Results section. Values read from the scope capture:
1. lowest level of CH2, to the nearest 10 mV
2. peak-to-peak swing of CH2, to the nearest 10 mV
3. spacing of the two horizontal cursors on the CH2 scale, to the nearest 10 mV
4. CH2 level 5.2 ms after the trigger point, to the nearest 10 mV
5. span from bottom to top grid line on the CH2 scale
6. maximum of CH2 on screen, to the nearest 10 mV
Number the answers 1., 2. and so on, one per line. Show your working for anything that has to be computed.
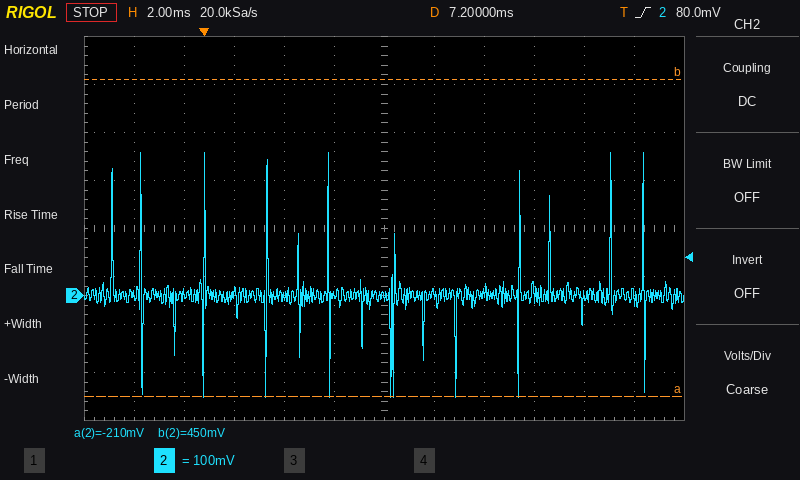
1. -210 mV
2. 300 mV − (-210 mV) = 510 mV
3. 660 mV
4. 0 mV
5. 800 mV
6. 300 mV
